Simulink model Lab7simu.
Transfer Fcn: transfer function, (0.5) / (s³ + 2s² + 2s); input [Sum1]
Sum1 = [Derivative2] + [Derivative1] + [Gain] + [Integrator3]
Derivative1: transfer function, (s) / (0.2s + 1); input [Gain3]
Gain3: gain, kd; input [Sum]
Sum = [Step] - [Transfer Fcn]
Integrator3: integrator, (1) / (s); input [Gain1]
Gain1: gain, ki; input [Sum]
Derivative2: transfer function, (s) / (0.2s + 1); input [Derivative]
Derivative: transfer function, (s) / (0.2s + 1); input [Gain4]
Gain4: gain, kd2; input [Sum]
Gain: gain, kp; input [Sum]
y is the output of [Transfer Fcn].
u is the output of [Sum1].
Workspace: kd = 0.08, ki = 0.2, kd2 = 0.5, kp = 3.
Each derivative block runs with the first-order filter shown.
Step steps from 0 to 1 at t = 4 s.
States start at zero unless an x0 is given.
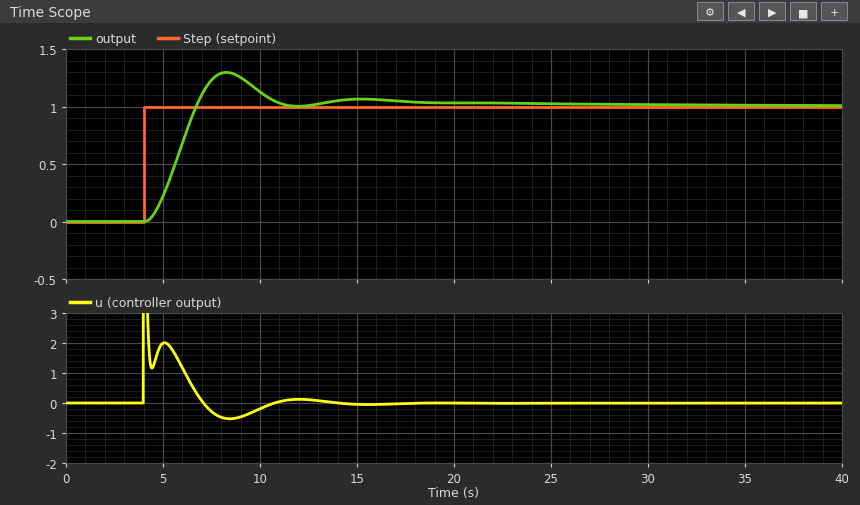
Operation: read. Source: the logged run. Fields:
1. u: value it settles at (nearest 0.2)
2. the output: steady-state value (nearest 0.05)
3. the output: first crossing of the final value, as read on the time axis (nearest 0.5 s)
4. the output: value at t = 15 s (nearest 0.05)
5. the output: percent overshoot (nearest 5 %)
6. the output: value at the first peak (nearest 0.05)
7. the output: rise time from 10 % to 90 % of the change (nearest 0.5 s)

0.0
1.00
6.5 s
1.05
30 %
1.30
2.0 s
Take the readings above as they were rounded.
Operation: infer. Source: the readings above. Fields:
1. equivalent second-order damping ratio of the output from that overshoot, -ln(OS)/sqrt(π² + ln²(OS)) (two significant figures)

0.36
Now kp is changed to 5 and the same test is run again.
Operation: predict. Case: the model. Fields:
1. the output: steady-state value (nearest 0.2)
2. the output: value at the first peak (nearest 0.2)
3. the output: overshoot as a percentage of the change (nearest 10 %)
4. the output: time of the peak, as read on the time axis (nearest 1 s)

1.0
1.4
50 %
7 s
